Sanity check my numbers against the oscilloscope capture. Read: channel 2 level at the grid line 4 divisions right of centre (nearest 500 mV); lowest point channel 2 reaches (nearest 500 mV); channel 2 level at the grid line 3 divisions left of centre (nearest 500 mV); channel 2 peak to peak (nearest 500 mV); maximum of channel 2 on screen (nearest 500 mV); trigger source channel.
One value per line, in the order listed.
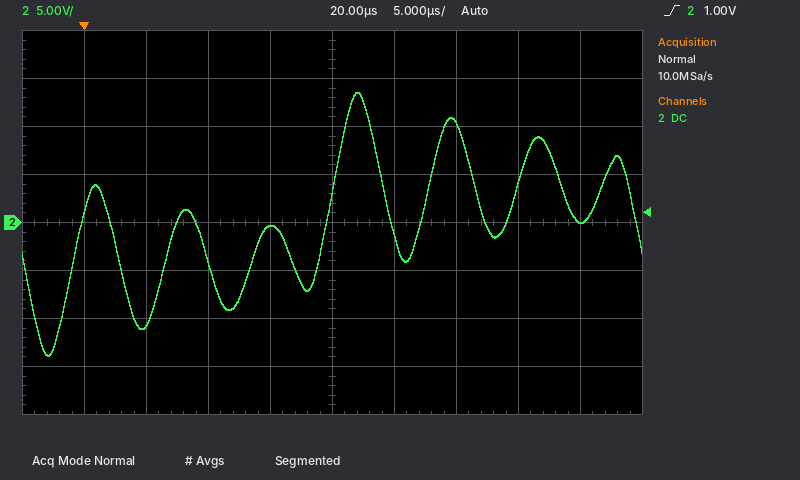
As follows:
0.0 V
-14.0 V
-10.5 V
27.5 V
13.5 V
channel 2
